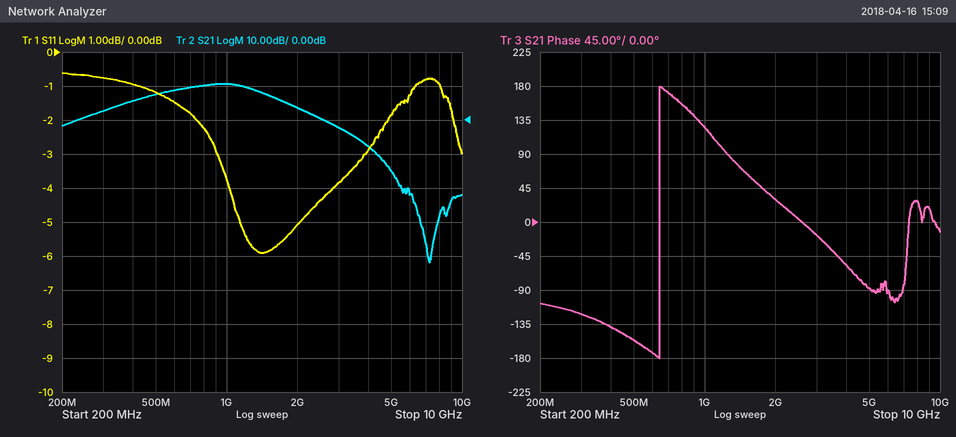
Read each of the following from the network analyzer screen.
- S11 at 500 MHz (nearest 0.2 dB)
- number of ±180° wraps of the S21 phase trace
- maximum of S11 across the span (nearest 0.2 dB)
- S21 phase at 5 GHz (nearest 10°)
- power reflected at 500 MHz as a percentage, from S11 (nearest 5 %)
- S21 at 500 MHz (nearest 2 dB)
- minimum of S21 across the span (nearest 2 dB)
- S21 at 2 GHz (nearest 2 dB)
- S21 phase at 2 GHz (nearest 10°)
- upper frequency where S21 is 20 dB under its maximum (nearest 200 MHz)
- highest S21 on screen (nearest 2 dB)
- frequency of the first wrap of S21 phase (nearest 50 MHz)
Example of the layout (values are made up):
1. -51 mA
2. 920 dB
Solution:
1. -1.2 dB
2. 1
3. -0.6 dB
4. -90°
5. 75 %
6. 8 dB
7. -42 dB
8. 4 dB
9. 30°
10. 4.2 GHz
11. 10 dB
12. 650 MHz
